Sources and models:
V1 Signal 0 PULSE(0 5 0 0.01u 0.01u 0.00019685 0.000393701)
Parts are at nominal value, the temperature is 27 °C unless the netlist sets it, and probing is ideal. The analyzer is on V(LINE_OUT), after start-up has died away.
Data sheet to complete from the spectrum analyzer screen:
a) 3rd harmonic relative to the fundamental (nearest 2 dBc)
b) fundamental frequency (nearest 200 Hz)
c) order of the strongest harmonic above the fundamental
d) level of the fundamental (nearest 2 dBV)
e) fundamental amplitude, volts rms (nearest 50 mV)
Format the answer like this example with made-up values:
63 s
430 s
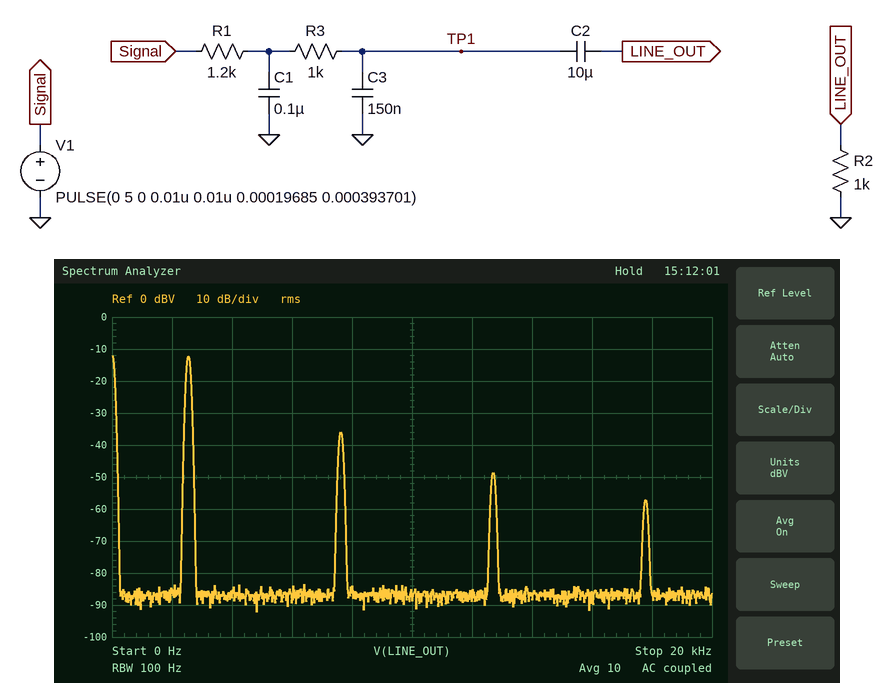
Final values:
-24 dBc
2.6 kHz
3
-12 dBV
250 mV
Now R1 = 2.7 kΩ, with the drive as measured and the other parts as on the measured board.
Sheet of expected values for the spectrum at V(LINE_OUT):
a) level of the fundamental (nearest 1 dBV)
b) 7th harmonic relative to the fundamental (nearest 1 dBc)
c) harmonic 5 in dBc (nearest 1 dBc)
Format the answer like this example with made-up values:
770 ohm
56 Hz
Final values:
-18 dBV
-46 dBc
-37 dBc
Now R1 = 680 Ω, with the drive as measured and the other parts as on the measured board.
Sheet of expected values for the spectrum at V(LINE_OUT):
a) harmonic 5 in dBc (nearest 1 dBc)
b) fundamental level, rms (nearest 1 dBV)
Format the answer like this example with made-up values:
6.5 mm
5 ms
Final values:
-35 dBc
-9 dBV
